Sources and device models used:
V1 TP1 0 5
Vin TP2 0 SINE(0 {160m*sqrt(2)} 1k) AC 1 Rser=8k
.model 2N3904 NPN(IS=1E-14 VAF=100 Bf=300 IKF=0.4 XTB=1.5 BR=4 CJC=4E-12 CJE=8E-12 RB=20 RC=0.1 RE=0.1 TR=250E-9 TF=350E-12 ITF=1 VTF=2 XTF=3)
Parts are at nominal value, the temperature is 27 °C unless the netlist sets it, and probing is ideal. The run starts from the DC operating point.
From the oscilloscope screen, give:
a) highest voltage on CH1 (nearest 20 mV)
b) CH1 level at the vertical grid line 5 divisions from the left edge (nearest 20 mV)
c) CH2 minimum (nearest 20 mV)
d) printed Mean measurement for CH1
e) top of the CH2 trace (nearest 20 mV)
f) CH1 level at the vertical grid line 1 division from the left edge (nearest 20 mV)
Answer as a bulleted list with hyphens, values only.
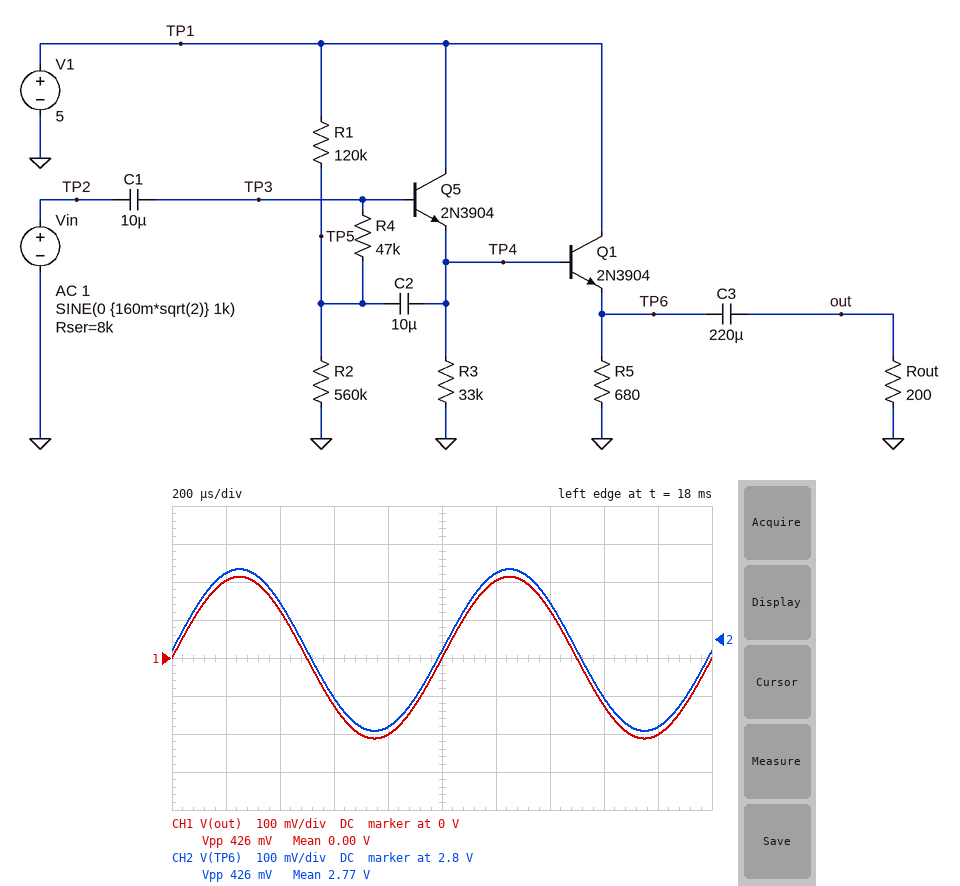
- 220 mV
- 0 V
- 2.56 V
- 0.00 V
- 2.98 V
- 200 mV
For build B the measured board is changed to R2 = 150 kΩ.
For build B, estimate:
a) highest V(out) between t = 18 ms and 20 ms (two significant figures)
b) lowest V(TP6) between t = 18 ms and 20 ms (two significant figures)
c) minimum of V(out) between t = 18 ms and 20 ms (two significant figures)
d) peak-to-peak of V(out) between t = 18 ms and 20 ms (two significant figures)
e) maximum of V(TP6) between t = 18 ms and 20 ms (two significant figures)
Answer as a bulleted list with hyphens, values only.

- 210 mV
- 1.3 V
- -200 mV
- 400 mV
- 1.7 V
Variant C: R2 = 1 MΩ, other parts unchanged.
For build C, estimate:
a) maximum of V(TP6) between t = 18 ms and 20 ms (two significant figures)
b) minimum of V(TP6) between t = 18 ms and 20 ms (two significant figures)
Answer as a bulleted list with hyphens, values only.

- 3.3 V
- 2.9 V
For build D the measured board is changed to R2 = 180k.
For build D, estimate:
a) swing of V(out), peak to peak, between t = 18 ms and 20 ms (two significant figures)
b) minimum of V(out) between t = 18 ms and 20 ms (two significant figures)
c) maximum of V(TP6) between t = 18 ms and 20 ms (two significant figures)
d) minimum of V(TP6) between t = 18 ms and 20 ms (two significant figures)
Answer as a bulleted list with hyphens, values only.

- 410 mV
- -200 mV
- 1.9 V
- 1.5 V
